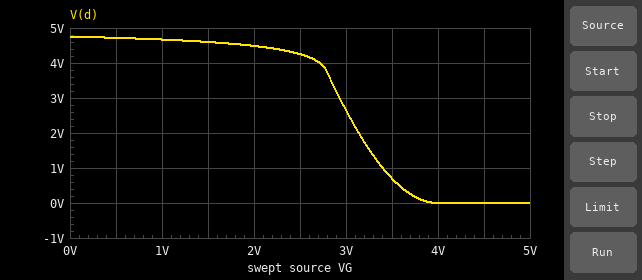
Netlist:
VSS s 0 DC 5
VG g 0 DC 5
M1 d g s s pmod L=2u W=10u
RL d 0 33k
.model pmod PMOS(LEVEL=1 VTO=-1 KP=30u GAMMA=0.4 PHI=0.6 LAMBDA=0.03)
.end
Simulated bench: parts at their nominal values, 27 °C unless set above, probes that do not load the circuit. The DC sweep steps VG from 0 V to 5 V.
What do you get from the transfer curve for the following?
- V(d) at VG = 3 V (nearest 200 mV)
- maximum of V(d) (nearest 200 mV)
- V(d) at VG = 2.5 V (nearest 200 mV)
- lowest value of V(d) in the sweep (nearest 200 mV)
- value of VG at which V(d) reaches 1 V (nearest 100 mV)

2.6 V
4.8 V
4.2 V
0 V
3.4 V
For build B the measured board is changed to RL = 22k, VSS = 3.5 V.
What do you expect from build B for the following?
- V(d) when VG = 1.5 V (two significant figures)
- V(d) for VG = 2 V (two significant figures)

1.7 V
450 mV
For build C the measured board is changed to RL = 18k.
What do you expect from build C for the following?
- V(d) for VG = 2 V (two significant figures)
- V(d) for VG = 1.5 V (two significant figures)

4.0 V
4.3 V
